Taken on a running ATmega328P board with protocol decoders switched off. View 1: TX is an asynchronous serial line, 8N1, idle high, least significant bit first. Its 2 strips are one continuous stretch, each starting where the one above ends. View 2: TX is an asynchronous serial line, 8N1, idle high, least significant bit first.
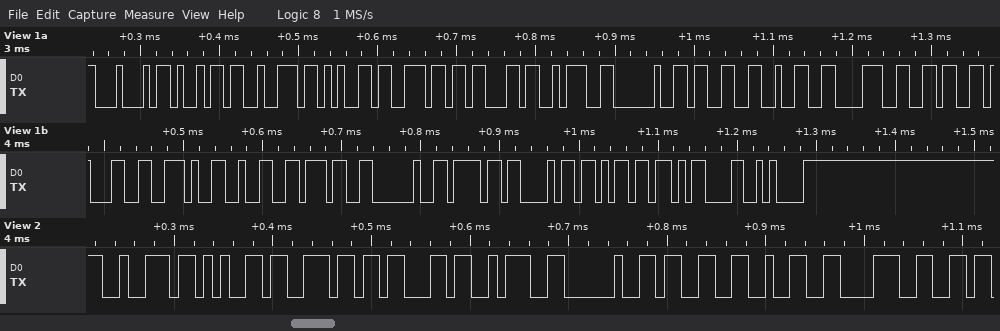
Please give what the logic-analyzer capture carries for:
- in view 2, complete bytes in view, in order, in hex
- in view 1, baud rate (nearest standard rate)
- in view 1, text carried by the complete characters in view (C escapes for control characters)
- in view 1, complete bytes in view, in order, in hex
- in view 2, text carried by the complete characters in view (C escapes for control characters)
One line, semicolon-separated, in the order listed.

0x72 0x65 0x6E 0x63 0x3A 0x20 0x33 0x32 0x38; 115200 baud; "Direnc: 32861.27 ohm\r\n"; 44 69 72 65 6E 63 3A 20 33 32 38 36 31 2E 32 37 20 6F 68 6D 0D 0A; "renc: 328"
